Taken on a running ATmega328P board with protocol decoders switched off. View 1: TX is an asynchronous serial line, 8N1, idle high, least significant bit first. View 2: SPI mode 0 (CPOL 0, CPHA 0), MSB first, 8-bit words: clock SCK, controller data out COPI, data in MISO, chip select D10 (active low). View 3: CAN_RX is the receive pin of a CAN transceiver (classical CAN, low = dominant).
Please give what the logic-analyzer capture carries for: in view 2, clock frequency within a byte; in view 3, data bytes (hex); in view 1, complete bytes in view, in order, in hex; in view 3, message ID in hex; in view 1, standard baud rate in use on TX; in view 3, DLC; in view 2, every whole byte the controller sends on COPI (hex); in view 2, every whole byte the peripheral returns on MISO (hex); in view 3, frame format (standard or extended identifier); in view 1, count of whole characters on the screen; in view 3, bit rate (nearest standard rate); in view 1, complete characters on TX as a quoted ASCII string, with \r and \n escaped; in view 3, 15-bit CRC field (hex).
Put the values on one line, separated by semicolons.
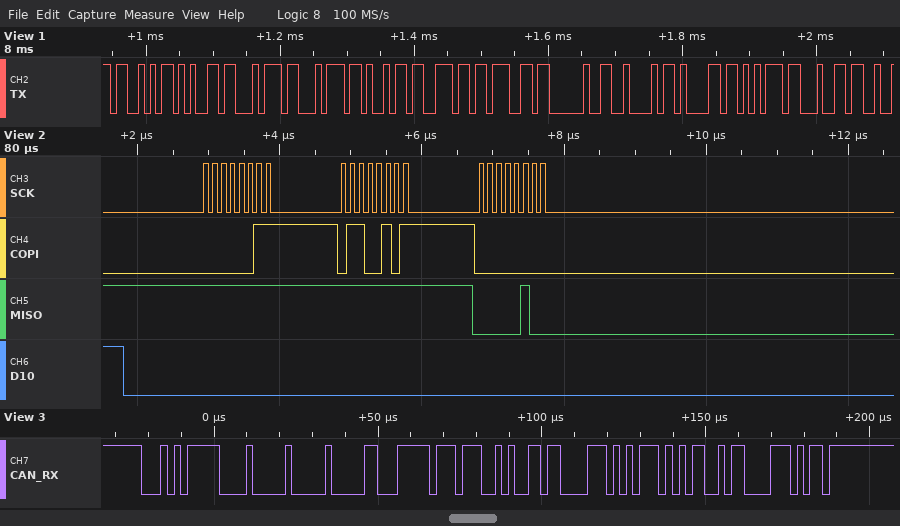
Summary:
8 MHz; 00 08 FF 72 9B 0E AE AC; 53 65 74 74 69 6E 67 20 42 61 75 64; 0x15F; 115200 baud; 8; 03 65 00; FF FF 04; standard; 12; 500 kbit/s; "Setting Baud"; 0x5875
